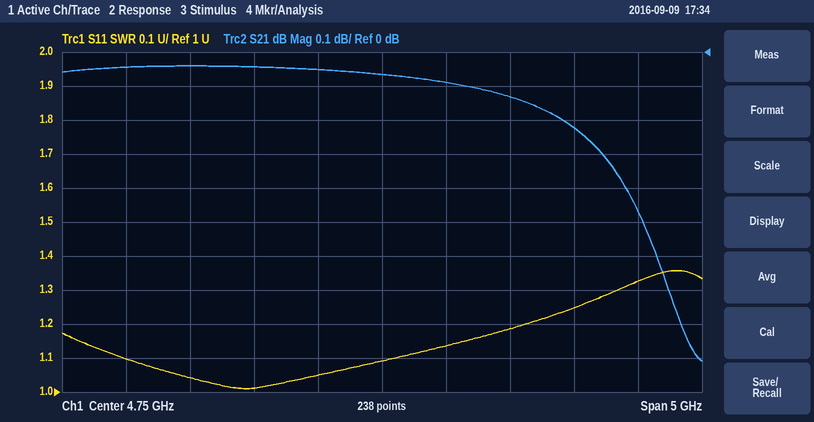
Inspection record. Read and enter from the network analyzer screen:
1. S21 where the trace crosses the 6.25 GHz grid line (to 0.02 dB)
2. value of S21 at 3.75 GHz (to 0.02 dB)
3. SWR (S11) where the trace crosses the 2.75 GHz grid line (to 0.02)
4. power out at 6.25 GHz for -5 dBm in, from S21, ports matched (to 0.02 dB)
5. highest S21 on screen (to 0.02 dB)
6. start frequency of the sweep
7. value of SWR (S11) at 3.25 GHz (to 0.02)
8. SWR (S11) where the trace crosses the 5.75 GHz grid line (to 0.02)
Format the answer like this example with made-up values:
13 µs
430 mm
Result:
-0.22 dB
-0.04 dB
1.10
-5.22 dBm
-0.04 dB
2.25 GHz
1.04
1.18
